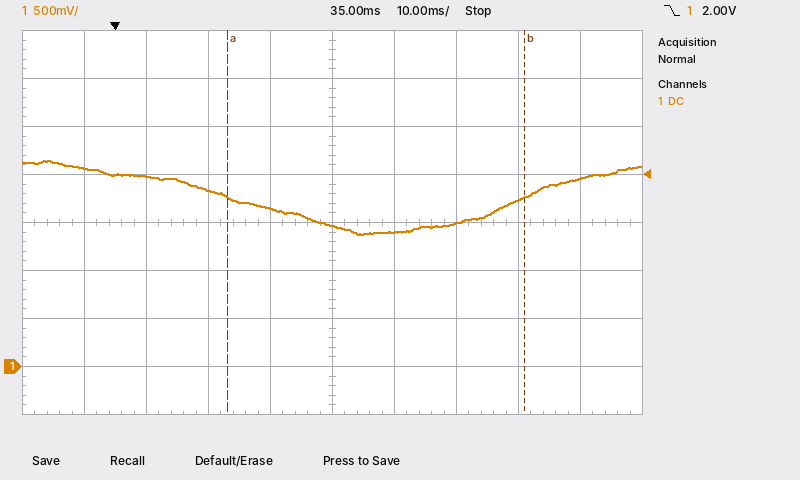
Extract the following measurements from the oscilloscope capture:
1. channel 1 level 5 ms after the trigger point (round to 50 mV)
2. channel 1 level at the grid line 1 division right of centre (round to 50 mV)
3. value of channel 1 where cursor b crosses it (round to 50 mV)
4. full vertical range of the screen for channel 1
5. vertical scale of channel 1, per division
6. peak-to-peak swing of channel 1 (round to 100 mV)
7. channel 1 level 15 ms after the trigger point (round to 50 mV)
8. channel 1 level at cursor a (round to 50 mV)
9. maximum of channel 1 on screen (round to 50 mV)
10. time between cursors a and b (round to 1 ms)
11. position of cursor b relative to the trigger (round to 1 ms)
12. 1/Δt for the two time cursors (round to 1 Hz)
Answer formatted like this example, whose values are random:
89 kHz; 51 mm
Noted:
2.00 V; 1.40 V; 1.75 V; 4 V; 500 mV; 800 mV; 1.85 V; 1.75 V; 2.15 V; 48 ms; +66 ms; 21 Hz
